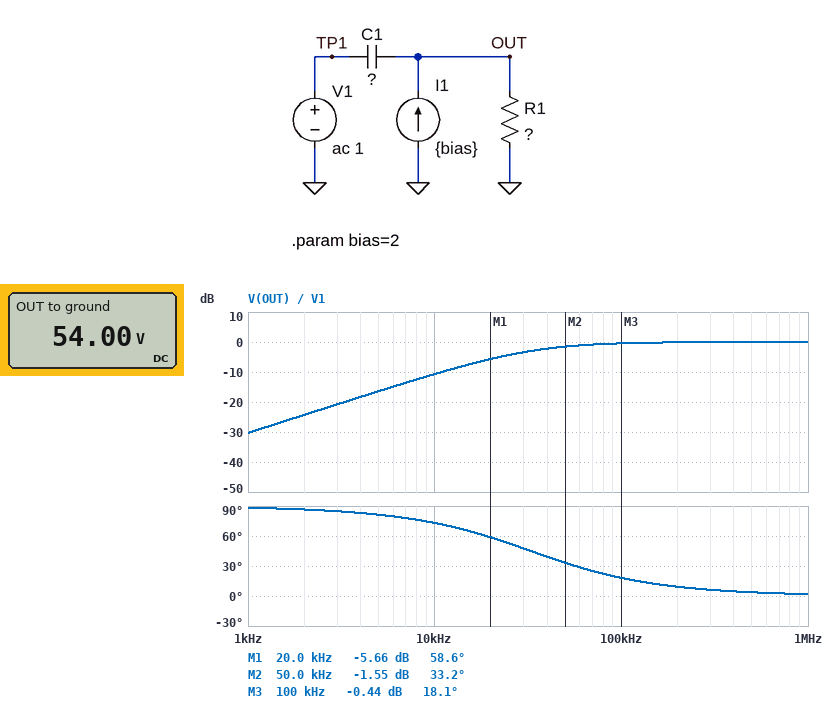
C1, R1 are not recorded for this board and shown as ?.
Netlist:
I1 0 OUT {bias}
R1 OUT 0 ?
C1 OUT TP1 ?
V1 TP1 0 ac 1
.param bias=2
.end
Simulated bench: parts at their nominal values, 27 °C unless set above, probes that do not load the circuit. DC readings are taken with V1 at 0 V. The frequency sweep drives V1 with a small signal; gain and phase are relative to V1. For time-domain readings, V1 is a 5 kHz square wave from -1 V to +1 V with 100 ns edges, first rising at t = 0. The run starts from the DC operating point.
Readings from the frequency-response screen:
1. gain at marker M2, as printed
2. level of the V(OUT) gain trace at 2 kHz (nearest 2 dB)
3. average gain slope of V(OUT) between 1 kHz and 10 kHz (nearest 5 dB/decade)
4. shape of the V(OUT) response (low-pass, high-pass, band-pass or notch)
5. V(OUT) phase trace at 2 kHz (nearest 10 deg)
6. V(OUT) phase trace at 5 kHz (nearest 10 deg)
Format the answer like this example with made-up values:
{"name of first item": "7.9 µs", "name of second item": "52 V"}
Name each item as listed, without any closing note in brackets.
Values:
{"gain at marker M2, as printed": "-1.55 dB", "level of the V(OUT) gain trace at 2 kHz": "-24 dB", "average gain slope of V(OUT) between 1 kHz and 10 kHz": "20 dB/decade", "shape of the V(OUT) response": "high-pass", "V(OUT) phase trace at 2 kHz": "90 deg", "V(OUT) phase trace at 5 kHz": "80 deg"}
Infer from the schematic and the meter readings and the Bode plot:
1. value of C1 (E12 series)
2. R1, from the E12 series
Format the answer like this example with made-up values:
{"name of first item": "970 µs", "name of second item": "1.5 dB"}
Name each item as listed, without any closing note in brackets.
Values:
{"value of C1": "180 nF", "R1, from the E12 series": "27 Ω"}
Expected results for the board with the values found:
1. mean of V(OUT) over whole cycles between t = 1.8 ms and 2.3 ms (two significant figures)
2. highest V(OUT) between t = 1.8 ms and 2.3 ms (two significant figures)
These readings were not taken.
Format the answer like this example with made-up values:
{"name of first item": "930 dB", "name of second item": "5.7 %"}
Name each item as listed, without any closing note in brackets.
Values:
{"mean of V(OUT) over whole cycles between t = 1.8 ms and 2.3 ms": "54 V", "highest V(OUT) between t = 1.8 ms and 2.3 ms": "56 V"}
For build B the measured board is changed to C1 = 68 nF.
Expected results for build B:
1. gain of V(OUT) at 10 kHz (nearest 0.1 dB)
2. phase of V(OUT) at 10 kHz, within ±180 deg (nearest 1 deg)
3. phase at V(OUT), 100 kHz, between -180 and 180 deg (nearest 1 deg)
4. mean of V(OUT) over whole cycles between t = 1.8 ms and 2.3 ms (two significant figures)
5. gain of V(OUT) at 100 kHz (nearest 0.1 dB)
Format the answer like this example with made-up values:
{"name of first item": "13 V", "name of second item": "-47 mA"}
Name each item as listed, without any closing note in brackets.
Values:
{"gain of V(OUT) at 10 kHz": "-18.8 dB", "phase of V(OUT) at 10 kHz, within ±180 deg": "83 deg", "phase at V(OUT), 100 kHz, between -180 and 180 deg": "41 deg", "mean of V(OUT) over whole cycles between t = 1.8 ms and 2.3 ms": "54 V", "gain of V(OUT) at 100 kHz": "-2.4 dB"}
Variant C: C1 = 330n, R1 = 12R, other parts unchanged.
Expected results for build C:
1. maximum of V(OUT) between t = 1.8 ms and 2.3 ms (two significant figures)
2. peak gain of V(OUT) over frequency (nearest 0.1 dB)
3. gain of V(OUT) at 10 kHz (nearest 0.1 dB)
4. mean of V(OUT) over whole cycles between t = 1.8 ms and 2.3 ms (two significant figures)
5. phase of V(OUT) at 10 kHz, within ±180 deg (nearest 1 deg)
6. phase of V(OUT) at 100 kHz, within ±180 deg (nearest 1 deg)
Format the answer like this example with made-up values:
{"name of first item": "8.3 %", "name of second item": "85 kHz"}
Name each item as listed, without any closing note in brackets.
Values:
{"maximum of V(OUT) between t = 1.8 ms and 2.3 ms": "26 V", "peak gain of V(OUT) over frequency": "0 dB", "gain of V(OUT) at 10 kHz": "-12.3 dB", "mean of V(OUT) over whole cycles between t = 1.8 ms and 2.3 ms": "24 V", "phase of V(OUT) at 10 kHz, within ±180 deg": "76 deg", "phase of V(OUT) at 100 kHz, within ±180 deg": "22 deg"}
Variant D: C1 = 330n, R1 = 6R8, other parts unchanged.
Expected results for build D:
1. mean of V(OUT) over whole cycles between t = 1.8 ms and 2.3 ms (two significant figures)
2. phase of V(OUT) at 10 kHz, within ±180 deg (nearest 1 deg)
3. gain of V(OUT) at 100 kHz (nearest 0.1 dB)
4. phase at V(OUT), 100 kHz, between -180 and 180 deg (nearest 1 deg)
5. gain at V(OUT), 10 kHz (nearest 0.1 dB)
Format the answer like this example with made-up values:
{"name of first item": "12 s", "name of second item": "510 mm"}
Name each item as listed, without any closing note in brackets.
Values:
{"mean of V(OUT) over whole cycles between t = 1.8 ms and 2.3 ms": "14 V", "phase of V(OUT) at 10 kHz, within ±180 deg": "82 deg", "gain of V(OUT) at 100 kHz": "-1.8 dB", "phase at V(OUT), 100 kHz, between -180 and 180 deg": "35 deg", "gain at V(OUT), 10 kHz": "-17.1 dB"}
